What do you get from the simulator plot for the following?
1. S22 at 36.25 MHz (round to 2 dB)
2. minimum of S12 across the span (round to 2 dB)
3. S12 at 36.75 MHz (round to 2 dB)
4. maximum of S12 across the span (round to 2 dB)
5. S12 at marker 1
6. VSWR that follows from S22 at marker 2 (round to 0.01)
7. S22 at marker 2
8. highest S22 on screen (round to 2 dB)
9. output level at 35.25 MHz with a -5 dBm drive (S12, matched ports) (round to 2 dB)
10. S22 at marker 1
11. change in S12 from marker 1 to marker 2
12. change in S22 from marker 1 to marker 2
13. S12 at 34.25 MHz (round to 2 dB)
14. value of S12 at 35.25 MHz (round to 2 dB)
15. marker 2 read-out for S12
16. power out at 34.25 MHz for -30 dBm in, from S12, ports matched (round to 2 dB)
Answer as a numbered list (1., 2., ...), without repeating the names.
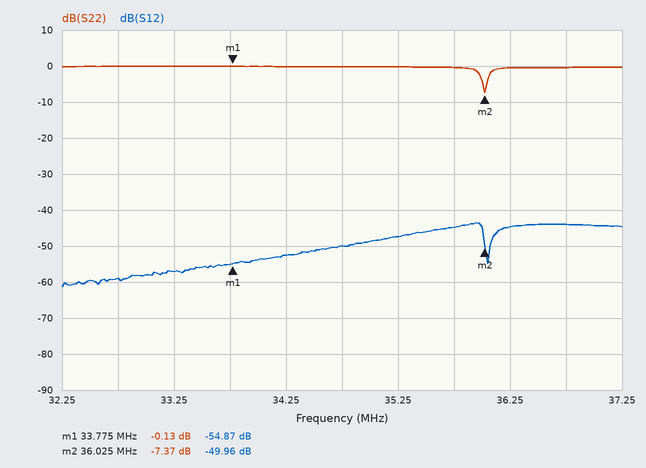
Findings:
1. 0 dB
2. -62 dB
3. -44 dB
4. -44 dB
5. -54.87 dB
6. 2.50
7. -7.37 dB
8. 0 dB
9. -52 dBm
10. -0.13 dB
11. 4.91 dB
12. -7.24 dB
13. -52 dB
14. -48 dB
15. -49.96 dB
16. -82 dBm
